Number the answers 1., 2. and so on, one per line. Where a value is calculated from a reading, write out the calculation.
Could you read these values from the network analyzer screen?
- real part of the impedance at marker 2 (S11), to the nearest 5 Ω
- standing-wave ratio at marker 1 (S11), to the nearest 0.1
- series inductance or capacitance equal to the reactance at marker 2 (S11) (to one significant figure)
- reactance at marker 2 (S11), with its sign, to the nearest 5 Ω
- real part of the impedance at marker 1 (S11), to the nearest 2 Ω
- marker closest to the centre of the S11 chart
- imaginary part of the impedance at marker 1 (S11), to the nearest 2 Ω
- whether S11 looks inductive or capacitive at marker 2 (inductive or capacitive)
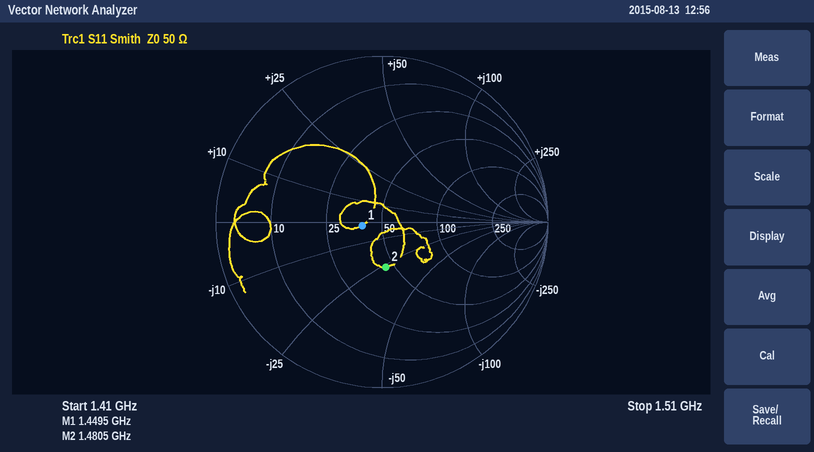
1. 45 Ω
2. 1.3
3. C = 1/(2π × 1.4805 GHz × 25 Ω) ≈ 4 pF
4. -25 Ω
5. 40 Ω
6. marker 1
7. -2 Ω
8. capacitive
